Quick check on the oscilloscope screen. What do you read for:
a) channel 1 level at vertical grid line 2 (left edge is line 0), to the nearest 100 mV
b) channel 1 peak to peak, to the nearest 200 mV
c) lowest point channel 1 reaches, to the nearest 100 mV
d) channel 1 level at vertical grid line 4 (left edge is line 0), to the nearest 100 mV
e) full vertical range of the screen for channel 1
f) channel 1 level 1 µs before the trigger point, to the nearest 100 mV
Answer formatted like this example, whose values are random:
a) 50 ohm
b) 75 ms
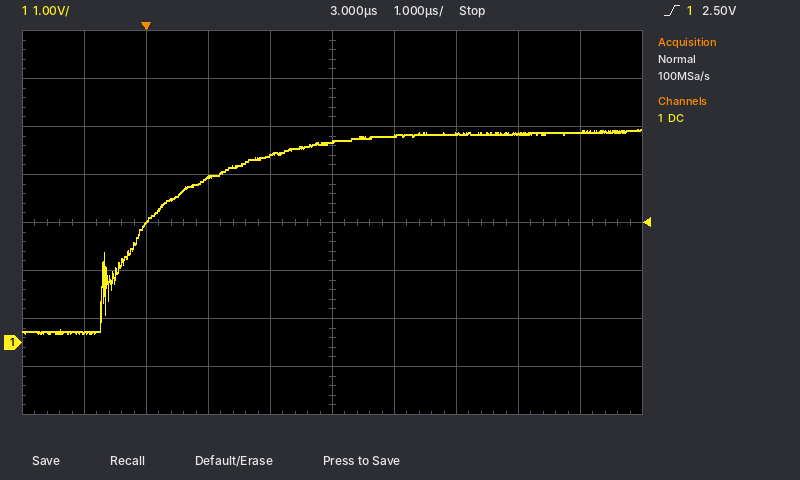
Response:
a) 2.5 V
b) 4.2 V
c) 200 mV
d) 3.9 V
e) 8 V
f) 200 mV
